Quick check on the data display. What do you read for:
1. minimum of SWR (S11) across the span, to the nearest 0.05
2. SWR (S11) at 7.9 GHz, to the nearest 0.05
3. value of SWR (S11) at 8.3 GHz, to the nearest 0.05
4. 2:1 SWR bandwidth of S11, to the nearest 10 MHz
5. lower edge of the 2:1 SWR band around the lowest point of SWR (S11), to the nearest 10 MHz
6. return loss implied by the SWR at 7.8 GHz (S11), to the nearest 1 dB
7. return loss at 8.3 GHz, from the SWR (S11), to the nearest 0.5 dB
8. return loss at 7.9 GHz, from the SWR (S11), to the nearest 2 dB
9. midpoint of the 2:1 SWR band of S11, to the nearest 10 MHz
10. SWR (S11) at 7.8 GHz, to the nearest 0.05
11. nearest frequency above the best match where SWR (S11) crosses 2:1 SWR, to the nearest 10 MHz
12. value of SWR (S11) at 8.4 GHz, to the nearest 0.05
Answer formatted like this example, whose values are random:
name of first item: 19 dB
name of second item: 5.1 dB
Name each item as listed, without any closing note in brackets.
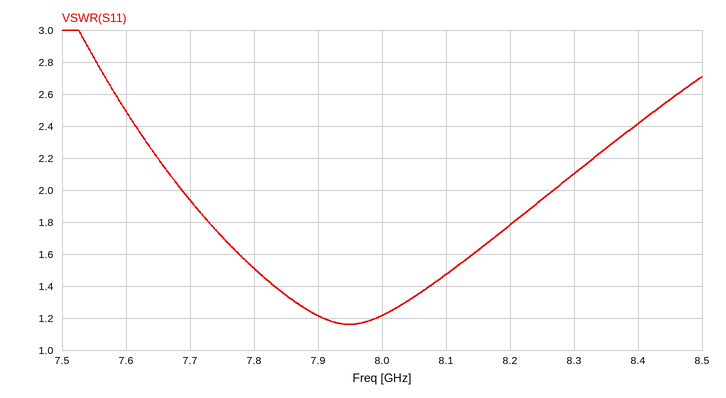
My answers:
minimum of SWR (S11) across the span, to the nearest 0.05: 1.15
SWR (S11) at 7.9 GHz, to the nearest 0.05: 1.20
value of SWR (S11) at 8.3 GHz, to the nearest 0.05: 2.10
2:1 SWR bandwidth of S11, to the nearest 10 MHz: 580 MHz
lower edge of the 2:1 SWR band around the lowest point of SWR (S11), to the nearest 10 MHz: 7.69 GHz
return loss implied by the SWR at 7.8 GHz (S11), to the nearest 1 dB: 14 dB
return loss at 8.3 GHz, from the SWR (S11), to the nearest 0.5 dB: 9.0 dB
return loss at 7.9 GHz, from the SWR (S11), to the nearest 2 dB: 20 dB
midpoint of the 2:1 SWR band of S11, to the nearest 10 MHz: 7.98 GHz
SWR (S11) at 7.8 GHz, to the nearest 0.05: 1.50
nearest frequency above the best match where SWR (S11) crosses 2:1 SWR, to the nearest 10 MHz: 8.27 GHz
value of SWR (S11) at 8.4 GHz, to the nearest 0.05: 2.40
